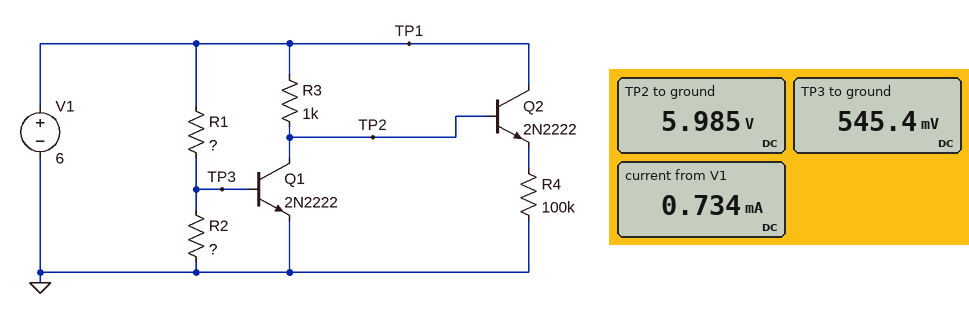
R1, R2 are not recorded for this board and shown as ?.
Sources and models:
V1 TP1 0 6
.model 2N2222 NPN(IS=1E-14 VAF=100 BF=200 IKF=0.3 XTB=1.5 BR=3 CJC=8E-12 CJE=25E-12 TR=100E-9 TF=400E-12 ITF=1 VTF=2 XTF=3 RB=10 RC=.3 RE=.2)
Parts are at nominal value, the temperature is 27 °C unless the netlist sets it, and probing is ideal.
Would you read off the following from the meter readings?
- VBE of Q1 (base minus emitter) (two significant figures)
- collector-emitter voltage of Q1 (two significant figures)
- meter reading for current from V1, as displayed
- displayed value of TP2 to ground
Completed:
550 mV
6.0 V
0.734 mA
5.985 V
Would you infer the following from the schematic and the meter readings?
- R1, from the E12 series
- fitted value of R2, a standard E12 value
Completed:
8.2 kΩ
820 Ω
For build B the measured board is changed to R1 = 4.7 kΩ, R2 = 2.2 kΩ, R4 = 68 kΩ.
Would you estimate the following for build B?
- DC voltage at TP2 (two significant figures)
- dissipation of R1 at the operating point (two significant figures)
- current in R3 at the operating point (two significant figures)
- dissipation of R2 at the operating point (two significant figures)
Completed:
40 mV
5.9 mW
6.0 mA
240 µW
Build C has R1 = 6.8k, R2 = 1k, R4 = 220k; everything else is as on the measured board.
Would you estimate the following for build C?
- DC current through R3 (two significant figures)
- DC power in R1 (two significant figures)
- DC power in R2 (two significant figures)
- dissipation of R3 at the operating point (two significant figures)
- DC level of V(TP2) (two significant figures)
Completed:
5.9 mA
4.1 mW
500 µW
35 mW
100 mV
